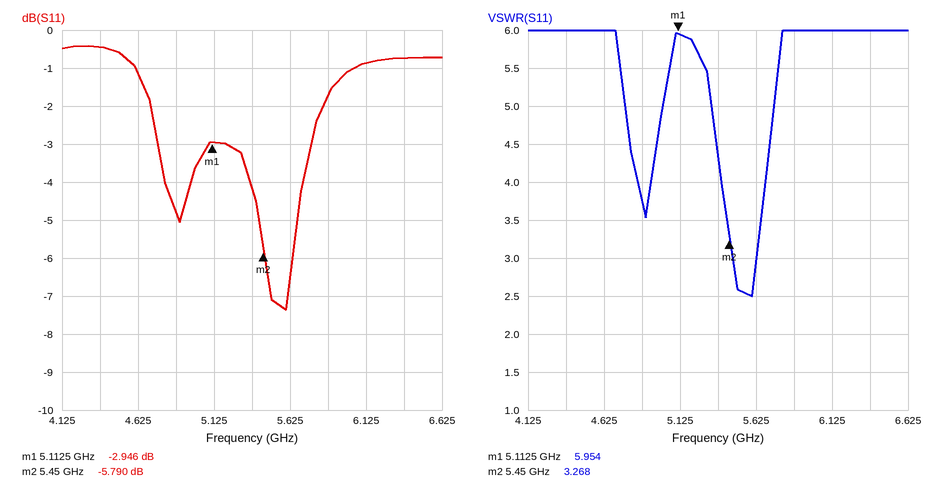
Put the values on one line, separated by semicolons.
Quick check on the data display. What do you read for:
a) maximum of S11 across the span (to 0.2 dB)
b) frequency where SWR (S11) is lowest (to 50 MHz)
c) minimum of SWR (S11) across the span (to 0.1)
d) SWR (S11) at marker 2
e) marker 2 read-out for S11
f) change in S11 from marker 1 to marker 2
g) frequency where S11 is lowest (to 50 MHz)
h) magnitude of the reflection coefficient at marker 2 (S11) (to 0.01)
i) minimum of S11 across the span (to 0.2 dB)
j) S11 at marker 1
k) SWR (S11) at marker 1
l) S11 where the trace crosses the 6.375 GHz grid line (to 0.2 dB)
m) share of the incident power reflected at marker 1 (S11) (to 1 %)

-0.4 dB; 5.60 GHz; 2.5; 3.268; -5.790 dB; -2.844 dB; 5.60 GHz; 0.51; -7.4 dB; -2.946 dB; 5.954; -0.8 dB; 51 %
